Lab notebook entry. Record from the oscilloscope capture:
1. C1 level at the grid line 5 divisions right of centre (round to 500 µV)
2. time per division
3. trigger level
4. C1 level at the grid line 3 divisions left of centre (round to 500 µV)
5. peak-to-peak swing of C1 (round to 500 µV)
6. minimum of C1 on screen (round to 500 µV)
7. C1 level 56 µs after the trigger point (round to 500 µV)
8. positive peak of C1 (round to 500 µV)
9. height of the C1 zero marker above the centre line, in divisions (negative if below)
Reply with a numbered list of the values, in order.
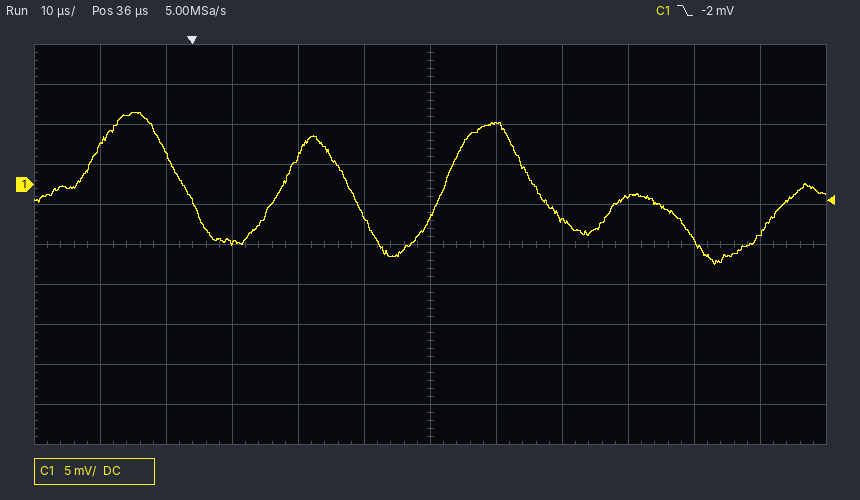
1. -6.0 mV
2. 10 µs
3. -2 mV
4. -7.5 mV
5. 19.0 mV
6. -10.0 mV
7. -4.5 mV
8. 9.0 mV
9. +1.5 div
